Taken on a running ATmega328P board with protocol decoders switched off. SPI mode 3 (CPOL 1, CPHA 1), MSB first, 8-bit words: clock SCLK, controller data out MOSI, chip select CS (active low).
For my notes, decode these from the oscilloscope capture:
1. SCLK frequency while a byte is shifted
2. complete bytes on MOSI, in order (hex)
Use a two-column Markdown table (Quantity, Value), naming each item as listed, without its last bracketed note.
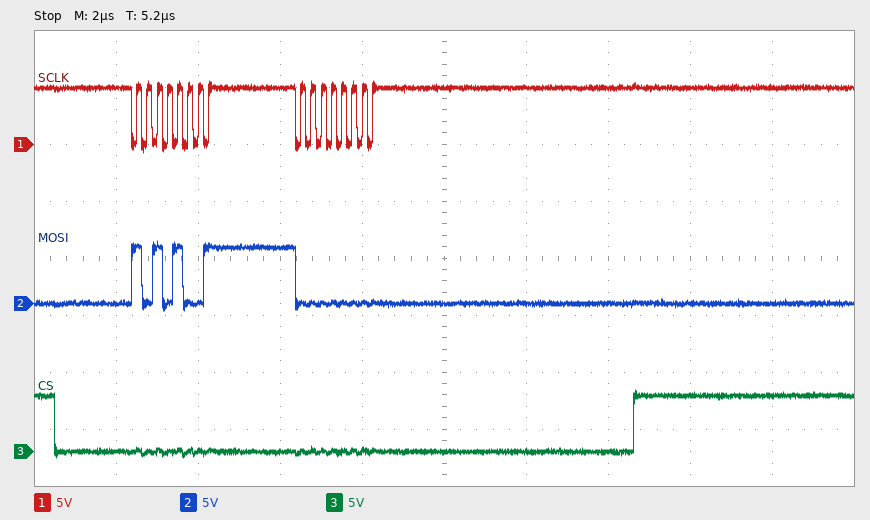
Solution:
| Quantity | Value |
|---|---|
| SCLK frequency while a byte is shifted | 4 MHz |
| complete bytes on MOSI, in order | A9 00 |
